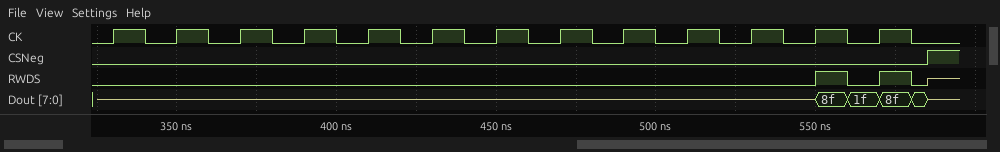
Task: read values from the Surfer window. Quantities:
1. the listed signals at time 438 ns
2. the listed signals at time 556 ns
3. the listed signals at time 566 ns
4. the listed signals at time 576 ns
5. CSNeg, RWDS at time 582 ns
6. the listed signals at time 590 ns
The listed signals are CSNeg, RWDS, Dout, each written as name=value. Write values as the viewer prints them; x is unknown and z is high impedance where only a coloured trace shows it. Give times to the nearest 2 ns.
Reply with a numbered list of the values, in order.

1. CSNeg=0, RWDS=0, Dout=z
2. CSNeg=0, RWDS=1, Dout=8f
3. CSNeg=0, RWDS=0, Dout=1f
4. CSNeg=0, RWDS=1, Dout=8f
5. CSNeg=0, RWDS=0
6. CSNeg=1, RWDS=z, Dout=z
